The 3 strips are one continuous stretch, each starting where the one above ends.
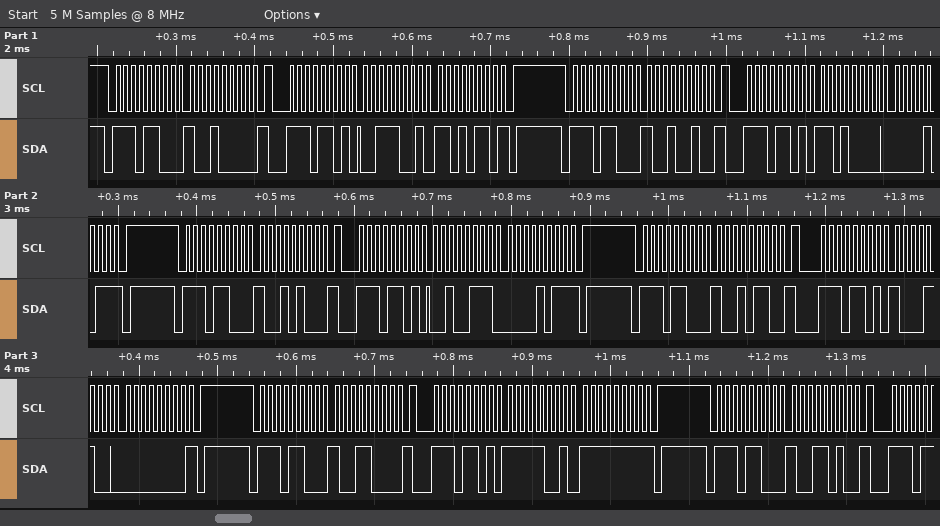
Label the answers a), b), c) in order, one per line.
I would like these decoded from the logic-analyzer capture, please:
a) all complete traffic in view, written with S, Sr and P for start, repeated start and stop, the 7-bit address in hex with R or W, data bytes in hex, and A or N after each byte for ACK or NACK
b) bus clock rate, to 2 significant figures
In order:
a) S 76W A 90 A Sr 76R A 39 A D6 N P S 76W A 92 A Sr 76R A D0 A 0B N P S 76W A 94 A Sr 76R A 27 A 0B N P S 76W A 96 A Sr 76R A 8C A 00 N P S 76W A 98 A Sr 76R A F9 A FF N P S 76W A 9A A
b) 100 kHz
